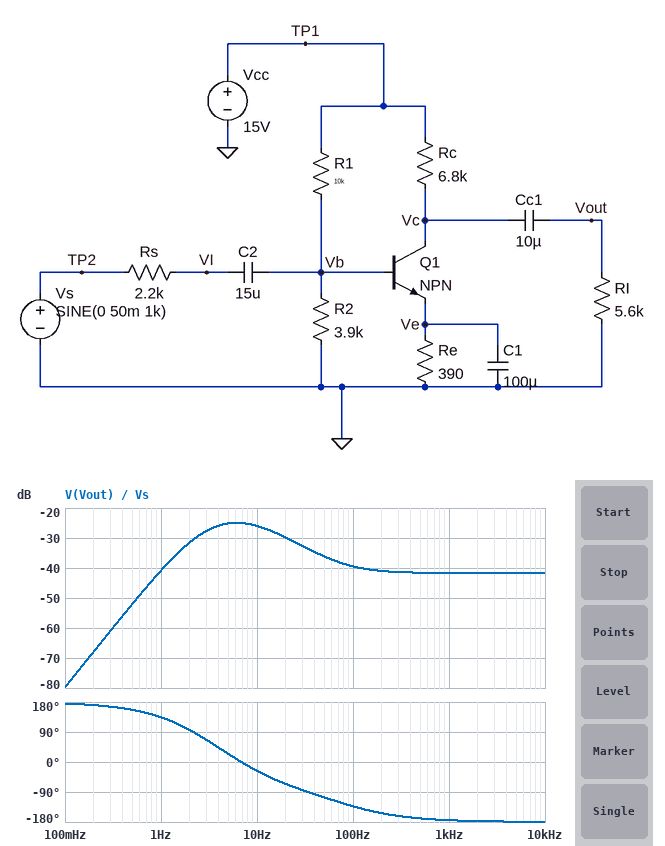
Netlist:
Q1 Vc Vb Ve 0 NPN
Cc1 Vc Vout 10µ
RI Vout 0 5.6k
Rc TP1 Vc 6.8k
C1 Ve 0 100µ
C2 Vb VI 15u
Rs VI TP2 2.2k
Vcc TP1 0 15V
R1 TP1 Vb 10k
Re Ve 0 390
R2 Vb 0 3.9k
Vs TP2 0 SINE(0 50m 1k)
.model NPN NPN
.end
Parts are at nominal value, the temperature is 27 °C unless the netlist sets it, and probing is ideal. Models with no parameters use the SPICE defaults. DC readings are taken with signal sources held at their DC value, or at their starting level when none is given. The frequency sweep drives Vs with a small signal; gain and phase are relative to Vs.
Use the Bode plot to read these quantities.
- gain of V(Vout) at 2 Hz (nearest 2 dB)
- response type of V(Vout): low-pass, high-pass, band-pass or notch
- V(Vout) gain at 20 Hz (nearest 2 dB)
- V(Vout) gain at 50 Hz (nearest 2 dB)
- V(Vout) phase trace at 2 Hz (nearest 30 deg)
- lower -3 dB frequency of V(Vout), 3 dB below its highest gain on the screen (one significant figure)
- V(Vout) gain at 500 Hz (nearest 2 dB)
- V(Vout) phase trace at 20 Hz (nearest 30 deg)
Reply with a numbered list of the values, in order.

1. -32 dB
2. band-pass
3. -30 dB
4. -36 dB
5. 90 deg
6. 3 Hz
7. -42 dB
8. -60 deg
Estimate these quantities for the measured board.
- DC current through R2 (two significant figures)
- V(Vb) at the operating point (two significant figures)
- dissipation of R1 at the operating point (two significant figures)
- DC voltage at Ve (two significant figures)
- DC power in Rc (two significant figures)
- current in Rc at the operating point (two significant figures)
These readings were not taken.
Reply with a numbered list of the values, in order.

1. 490 µA
2. 1.9 V
3. 17 mW
4. 1.1 V
5. 28 mW
6. 2.0 mA
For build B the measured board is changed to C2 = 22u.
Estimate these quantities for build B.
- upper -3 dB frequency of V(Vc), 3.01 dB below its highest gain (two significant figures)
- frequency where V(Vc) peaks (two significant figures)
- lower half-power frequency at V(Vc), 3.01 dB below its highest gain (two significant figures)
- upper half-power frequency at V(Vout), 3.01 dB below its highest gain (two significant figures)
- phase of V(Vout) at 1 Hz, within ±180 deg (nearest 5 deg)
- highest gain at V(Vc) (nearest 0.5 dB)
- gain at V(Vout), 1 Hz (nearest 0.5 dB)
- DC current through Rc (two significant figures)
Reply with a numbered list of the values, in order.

1. 11 Hz
2. 4.0 Hz
3. 1.5 Hz
4. 13 Hz
5. 130 deg
6. -22.5 dB
7. -38.0 dB
8. 2.0 mA
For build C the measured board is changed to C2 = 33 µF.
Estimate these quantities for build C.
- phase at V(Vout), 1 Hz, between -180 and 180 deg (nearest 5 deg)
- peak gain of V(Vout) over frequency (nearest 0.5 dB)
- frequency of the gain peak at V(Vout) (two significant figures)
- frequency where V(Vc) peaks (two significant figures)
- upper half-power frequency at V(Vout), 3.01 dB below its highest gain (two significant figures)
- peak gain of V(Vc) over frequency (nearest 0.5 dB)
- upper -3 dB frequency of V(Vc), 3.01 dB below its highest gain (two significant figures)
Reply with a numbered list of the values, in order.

1. 120 deg
2. -23.0 dB
3. 4.8 Hz
4. 3.2 Hz
5. 12 Hz
6. -21.5 dB
7. 9.2 Hz
